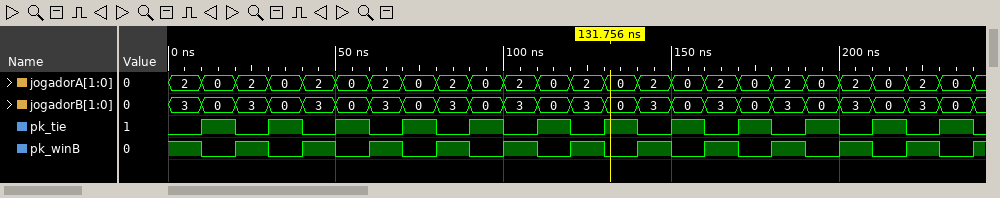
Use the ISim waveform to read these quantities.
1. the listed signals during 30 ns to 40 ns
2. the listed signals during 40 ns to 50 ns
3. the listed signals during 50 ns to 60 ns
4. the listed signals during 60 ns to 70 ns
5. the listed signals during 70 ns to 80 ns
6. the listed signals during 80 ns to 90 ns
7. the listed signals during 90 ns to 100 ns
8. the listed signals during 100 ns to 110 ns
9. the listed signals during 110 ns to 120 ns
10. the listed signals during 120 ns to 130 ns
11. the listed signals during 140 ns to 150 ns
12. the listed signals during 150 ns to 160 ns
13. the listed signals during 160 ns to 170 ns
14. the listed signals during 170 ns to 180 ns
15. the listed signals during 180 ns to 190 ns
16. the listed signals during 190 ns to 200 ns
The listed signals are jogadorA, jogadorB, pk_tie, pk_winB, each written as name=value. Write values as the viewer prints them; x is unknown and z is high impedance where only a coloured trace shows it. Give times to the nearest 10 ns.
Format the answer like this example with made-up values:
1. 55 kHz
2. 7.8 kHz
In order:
1. jogadorA=0, jogadorB=0, pk_tie=1, pk_winB=0
2. jogadorA=2, jogadorB=3, pk_tie=0, pk_winB=1
3. jogadorA=0, jogadorB=0, pk_tie=1, pk_winB=0
4. jogadorA=2, jogadorB=3, pk_tie=0, pk_winB=1
5. jogadorA=0, jogadorB=0, pk_tie=1, pk_winB=0
6. jogadorA=2, jogadorB=3, pk_tie=0, pk_winB=1
7. jogadorA=0, jogadorB=0, pk_tie=1, pk_winB=0
8. jogadorA=2, jogadorB=3, pk_tie=0, pk_winB=1
9. jogadorA=0, jogadorB=0, pk_tie=1, pk_winB=0
10. jogadorA=2, jogadorB=3, pk_tie=0, pk_winB=1
11. jogadorA=2, jogadorB=3, pk_tie=0, pk_winB=1
12. jogadorA=0, jogadorB=0, pk_tie=1, pk_winB=0
13. jogadorA=2, jogadorB=3, pk_tie=0, pk_winB=1
14. jogadorA=0, jogadorB=0, pk_tie=1, pk_winB=0
15. jogadorA=2, jogadorB=3, pk_tie=0, pk_winB=1
16. jogadorA=0, jogadorB=0, pk_tie=1, pk_winB=0
